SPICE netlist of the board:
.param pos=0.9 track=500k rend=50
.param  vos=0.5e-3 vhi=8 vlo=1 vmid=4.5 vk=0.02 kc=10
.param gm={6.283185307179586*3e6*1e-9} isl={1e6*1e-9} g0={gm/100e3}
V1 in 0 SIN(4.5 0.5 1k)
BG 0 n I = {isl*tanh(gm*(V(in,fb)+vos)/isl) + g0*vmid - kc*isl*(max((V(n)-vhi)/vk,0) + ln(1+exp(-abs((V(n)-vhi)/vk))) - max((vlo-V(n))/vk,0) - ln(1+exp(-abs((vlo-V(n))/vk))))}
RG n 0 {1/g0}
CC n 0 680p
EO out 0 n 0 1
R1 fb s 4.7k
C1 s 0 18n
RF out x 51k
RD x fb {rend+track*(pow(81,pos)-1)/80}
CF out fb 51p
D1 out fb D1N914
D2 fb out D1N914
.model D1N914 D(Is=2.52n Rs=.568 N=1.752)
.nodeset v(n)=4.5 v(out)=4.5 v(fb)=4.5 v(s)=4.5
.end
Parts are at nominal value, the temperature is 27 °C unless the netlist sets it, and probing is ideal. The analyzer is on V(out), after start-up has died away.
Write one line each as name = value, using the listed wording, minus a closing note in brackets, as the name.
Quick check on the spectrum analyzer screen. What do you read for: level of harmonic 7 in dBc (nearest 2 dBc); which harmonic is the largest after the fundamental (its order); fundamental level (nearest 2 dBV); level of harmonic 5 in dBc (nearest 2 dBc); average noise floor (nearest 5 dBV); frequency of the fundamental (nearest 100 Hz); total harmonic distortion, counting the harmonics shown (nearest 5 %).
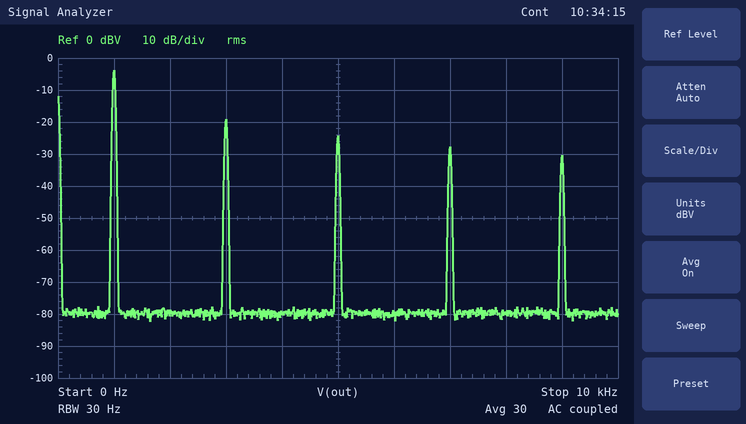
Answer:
level of harmonic 7 in dBc = -24 dBc
which harmonic is the largest after the fundamental = 3
fundamental level = -4 dBV
level of harmonic 5 in dBc = -20 dBc
average noise floor = -80 dBV
frequency of the fundamental = 1.0 kHz
total harmonic distortion, counting the harmonics shown = 20 %
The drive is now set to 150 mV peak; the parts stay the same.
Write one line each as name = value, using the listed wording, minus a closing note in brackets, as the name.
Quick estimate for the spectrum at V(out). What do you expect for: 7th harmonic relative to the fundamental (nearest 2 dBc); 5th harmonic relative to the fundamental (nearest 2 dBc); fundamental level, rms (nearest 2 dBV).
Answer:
7th harmonic relative to the fundamental = -22 dBc
5th harmonic relative to the fundamental = -18 dBc
fundamental level, rms = -8 dBV
